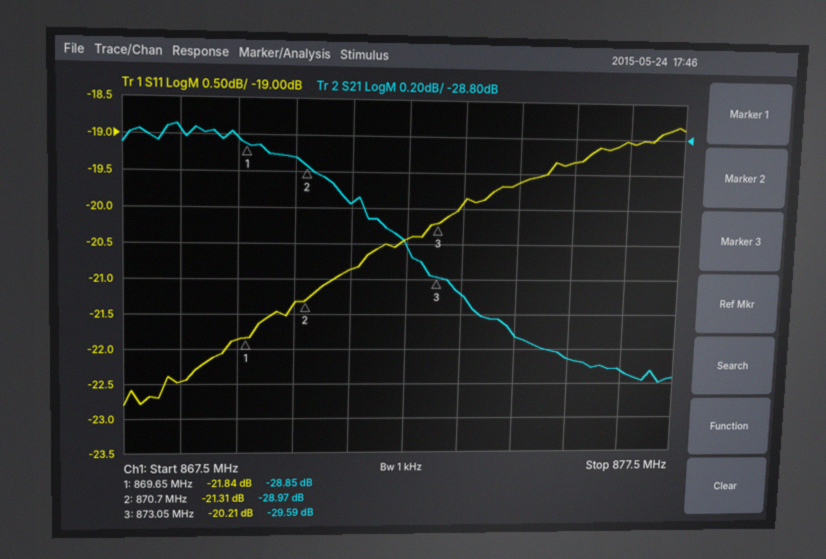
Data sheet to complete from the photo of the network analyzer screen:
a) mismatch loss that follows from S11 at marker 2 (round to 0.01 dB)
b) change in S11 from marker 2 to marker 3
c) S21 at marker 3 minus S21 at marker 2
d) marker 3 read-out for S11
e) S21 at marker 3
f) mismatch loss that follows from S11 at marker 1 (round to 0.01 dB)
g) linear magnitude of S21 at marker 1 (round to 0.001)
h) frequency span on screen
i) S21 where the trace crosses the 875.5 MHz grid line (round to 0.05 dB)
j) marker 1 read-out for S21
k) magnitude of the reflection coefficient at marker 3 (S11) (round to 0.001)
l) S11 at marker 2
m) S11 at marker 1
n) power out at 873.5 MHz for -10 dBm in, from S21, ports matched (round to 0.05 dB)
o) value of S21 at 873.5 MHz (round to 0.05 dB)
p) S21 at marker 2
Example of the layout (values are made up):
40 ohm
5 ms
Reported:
0.03 dB
1.10 dB
-0.62 dB
-20.21 dB
-29.59 dB
0.03 dB
0.036
10 MHz
-30.05 dB
-28.85 dB
0.098
-21.31 dB
-21.84 dB
-39.70 dBm
-29.70 dB
-28.97 dB
